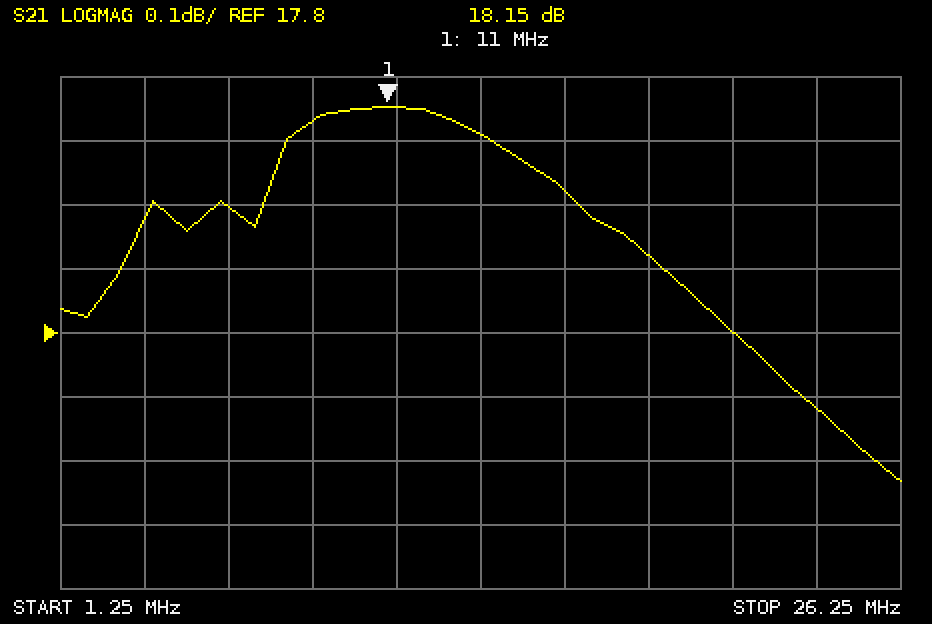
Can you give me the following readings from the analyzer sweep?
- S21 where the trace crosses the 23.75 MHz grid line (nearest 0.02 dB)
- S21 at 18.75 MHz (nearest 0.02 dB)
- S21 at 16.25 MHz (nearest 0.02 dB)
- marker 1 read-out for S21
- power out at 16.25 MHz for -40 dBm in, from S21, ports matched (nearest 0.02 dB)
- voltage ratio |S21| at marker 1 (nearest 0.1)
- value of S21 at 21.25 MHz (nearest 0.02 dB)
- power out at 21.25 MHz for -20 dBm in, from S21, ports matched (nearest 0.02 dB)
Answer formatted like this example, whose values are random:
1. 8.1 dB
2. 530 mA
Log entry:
1. 17.68 dB
2. 17.92 dB
3. 18.02 dB
4. 18.15 dB
5. -21.98 dBm
6. 8.1
7. 17.80 dB
8. -2.20 dBm
